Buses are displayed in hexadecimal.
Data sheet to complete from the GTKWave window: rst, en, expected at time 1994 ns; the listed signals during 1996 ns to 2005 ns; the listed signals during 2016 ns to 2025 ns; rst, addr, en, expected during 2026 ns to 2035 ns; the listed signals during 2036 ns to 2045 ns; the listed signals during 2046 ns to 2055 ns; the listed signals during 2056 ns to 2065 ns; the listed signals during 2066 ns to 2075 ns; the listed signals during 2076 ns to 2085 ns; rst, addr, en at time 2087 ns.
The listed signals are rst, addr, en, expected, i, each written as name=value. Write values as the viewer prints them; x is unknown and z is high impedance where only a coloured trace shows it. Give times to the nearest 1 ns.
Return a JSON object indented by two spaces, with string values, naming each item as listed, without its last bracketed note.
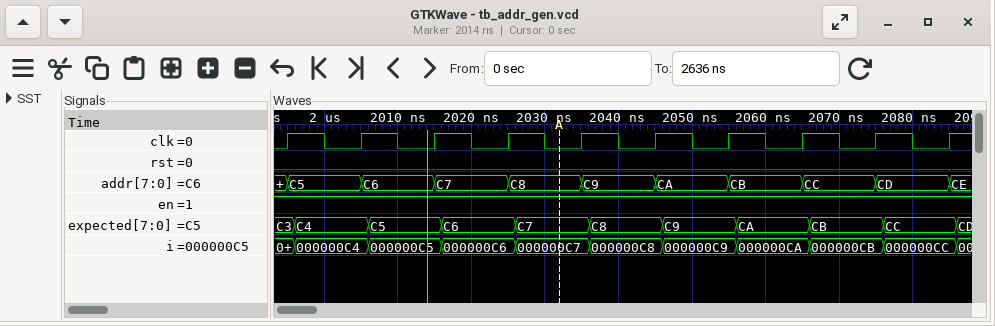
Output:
{
  "rst, en, expected at time 1994 ns": "rst=0, en=1, expected=C3",
  "the listed signals during 1996 ns to 2005 ns": "rst=0, addr=C5, en=1, expected=C4, i=000000C4",
  "the listed signals during 2016 ns to 2025 ns": "rst=0, addr=C7, en=1, expected=C6, i=000000C6",
  "rst, addr, en, expected during 2026 ns to 2035 ns": "rst=0, addr=C8, en=1, expected=C7",
  "the listed signals during 2036 ns to 2045 ns": "rst=0, addr=C9, en=1, expected=C8, i=000000C8",
  "the listed signals during 2046 ns to 2055 ns": "rst=0, addr=CA, en=1, expected=C9, i=000000C9",
  "the listed signals during 2056 ns to 2065 ns": "rst=0, addr=CB, en=1, expected=CA, i=000000CA",
  "the listed signals during 2066 ns to 2075 ns": "rst=0, addr=CC, en=1, expected=CB, i=000000CB",
  "the listed signals during 2076 ns to 2085 ns": "rst=0, addr=CD, en=1, expected=CC, i=000000CC",
  "rst, addr, en at time 2087 ns": "rst=0, addr=CE, en=1"
}
